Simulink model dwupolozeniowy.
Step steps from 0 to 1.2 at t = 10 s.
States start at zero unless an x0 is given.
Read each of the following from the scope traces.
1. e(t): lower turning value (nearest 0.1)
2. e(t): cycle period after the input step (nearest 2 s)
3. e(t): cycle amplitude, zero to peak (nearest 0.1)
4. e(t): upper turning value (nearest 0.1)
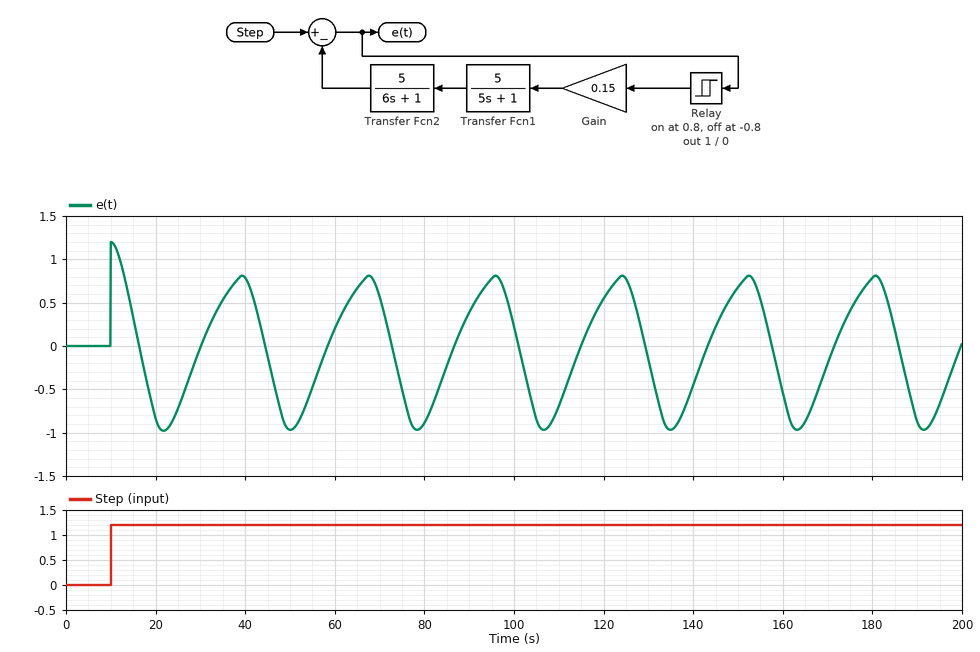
-1.0
28 s
0.9
0.8
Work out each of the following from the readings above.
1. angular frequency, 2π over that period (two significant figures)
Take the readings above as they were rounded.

0.22 rad/s
